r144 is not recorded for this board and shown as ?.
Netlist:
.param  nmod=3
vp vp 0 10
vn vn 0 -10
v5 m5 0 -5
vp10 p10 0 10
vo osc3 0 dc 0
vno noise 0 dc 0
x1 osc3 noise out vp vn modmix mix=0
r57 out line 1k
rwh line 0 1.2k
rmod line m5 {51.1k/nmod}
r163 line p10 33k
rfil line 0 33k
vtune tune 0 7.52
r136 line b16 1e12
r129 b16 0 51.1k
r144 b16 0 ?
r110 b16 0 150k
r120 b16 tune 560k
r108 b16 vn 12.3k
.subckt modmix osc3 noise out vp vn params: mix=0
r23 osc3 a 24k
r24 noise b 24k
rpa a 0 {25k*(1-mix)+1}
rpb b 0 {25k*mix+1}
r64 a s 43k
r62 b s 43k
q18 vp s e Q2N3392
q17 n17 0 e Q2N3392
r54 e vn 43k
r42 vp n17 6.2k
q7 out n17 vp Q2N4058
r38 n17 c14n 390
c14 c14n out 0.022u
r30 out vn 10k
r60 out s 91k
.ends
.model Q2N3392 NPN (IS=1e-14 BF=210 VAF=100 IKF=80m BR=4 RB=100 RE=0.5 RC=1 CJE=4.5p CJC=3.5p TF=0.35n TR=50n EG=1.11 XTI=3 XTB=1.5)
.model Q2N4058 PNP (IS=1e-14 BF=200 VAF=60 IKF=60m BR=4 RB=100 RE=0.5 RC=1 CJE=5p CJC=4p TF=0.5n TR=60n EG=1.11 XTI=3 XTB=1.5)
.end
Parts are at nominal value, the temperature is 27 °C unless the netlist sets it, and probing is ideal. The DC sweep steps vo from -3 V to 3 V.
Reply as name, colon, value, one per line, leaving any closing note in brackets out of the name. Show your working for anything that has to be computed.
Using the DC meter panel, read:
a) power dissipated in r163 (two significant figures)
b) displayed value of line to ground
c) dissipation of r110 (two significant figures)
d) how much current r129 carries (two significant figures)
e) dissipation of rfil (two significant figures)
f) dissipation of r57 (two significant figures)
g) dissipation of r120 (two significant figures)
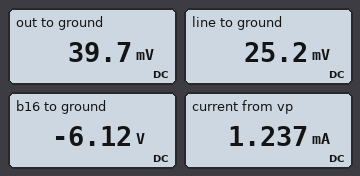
power dissipated in r163: (10 V - 25.2 mV)^2 / 33 kΩ = 3.0 mW
displayed value of line to ground: 25.2 mV
dissipation of r110: (0 V - (-6.12 V))^2 / 150 kΩ = 250 µW
how much current r129 carries: (0 V - (-6.12 V)) / 51.1 kΩ = 120 µA
dissipation of rfil: (25.2 mV)^2 / 33 kΩ = 19 nW
dissipation of r57: (39.7 mV - 25.2 mV)^2 / 1 kΩ = 210 nW
dissipation of r120: (7.52 V - (-6.12 V))^2 / 560 kΩ = 330 µW
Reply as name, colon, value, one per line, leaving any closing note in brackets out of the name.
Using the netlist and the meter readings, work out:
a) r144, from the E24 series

r144, from the E24 series: 47 kΩ
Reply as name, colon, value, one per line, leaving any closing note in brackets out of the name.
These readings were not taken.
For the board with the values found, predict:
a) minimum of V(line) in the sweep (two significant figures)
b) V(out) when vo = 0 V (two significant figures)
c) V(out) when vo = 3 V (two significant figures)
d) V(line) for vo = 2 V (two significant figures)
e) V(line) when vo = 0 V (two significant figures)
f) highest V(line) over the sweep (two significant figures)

minimum of V(line) in the sweep: -850 mV
V(out) when vo = 0 V: 40 mV
V(out) when vo = 3 V: -1.7 V
V(line) for vo = 2 V: -810 mV
V(line) when vo = 0 V: 25 mV
highest V(line) over the sweep: 1.3 V
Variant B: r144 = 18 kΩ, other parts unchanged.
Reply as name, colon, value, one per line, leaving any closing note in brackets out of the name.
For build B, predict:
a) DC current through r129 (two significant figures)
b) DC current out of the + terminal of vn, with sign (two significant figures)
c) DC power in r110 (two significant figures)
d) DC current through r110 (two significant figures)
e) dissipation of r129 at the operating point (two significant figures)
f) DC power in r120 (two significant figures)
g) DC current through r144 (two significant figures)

DC current through r129: 95 µA
DC current out of the + terminal of vn, with sign: -1.6 mA
DC power in r110: 160 µW
DC current through r110: 32 µA
dissipation of r129 at the operating point: 460 µW
DC power in r120: 270 µW
DC current through r144: 270 µA
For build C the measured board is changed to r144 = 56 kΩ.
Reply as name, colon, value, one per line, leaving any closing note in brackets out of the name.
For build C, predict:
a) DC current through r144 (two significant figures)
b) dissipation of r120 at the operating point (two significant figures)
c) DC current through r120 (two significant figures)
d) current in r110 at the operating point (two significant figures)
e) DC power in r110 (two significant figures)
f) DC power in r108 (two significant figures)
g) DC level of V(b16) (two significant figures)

DC current through r144: 110 µA
dissipation of r120 at the operating point: 340 µW
DC current through r120: 25 µA
current in r110 at the operating point: 42 µA
DC power in r110: 260 µW
DC power in r108: 1.1 mW
DC level of V(b16): -6.3 V
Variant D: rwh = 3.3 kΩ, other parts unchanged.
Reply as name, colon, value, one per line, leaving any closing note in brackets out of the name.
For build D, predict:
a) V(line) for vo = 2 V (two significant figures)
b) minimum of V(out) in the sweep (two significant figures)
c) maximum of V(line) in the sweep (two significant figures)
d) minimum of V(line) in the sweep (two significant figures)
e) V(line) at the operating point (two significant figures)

V(line) for vo = 2 V: -1.1 V
minimum of V(out) in the sweep: -2.4 V
maximum of V(line) in the sweep: 1.8 V
minimum of V(line) in the sweep: -1.7 V
V(line) at the operating point: 35 mV
